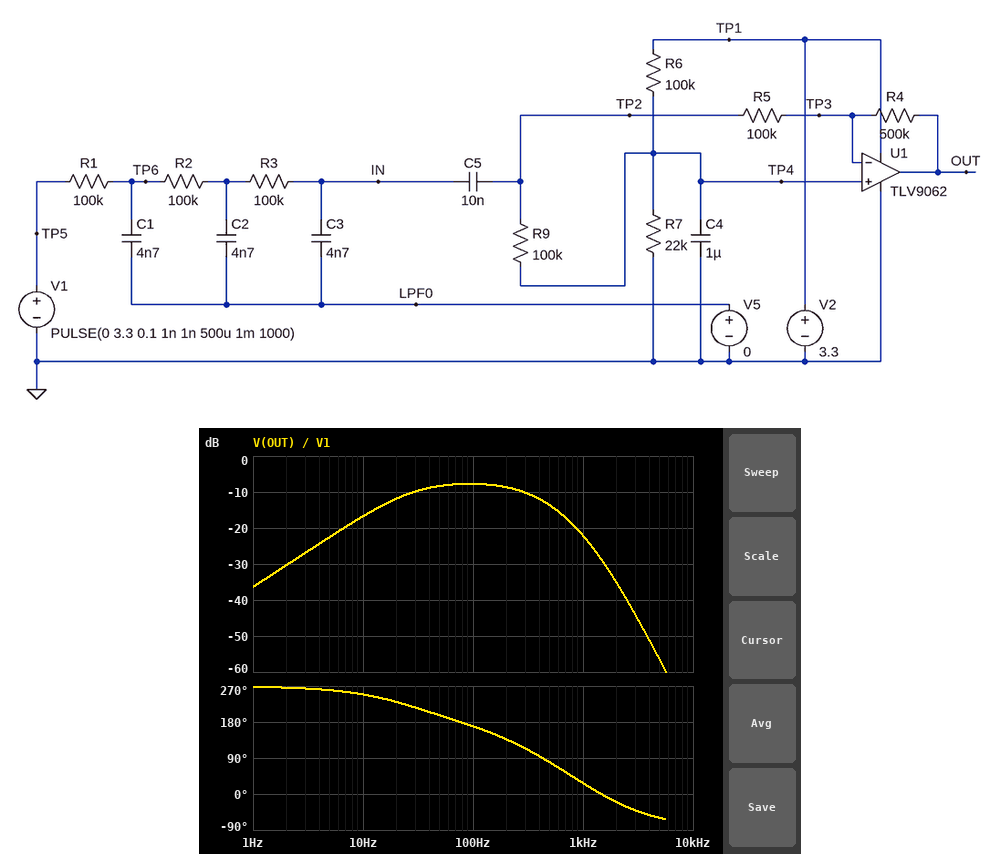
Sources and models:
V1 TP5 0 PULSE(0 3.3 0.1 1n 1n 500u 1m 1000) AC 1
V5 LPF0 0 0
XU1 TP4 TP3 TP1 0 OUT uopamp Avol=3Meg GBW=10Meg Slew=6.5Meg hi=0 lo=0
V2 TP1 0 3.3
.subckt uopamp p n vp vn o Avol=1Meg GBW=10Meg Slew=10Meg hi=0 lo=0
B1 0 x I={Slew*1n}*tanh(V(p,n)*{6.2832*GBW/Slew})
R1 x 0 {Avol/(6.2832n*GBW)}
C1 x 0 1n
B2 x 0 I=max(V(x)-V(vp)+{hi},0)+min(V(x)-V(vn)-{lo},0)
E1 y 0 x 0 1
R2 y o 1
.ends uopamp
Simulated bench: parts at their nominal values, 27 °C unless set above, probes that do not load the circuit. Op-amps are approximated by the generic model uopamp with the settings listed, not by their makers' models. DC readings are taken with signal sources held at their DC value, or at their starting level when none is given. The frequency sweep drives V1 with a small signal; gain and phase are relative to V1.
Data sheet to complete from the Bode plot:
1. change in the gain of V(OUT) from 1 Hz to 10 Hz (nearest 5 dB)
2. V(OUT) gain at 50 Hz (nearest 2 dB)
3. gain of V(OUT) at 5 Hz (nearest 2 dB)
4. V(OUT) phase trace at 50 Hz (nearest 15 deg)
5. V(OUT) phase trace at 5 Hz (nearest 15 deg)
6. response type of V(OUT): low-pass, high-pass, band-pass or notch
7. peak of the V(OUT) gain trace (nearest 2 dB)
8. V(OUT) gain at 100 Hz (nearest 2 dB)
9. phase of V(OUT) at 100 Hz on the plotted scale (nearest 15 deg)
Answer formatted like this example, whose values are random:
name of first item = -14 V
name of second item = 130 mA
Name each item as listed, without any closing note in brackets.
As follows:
change in the gain of V(OUT) from 1 Hz to 10 Hz = 20 dB
V(OUT) gain at 50 Hz = -8 dB
gain of V(OUT) at 5 Hz = -22 dB
V(OUT) phase trace at 50 Hz = 195 deg
V(OUT) phase trace at 5 Hz = 255 deg
response type of V(OUT): low-pass, high-pass, band-pass or notch = band-pass
peak of the V(OUT) gain trace = -8 dB
V(OUT) gain at 100 Hz = -8 dB
phase of V(OUT) at 100 Hz on the plotted scale = 165 deg
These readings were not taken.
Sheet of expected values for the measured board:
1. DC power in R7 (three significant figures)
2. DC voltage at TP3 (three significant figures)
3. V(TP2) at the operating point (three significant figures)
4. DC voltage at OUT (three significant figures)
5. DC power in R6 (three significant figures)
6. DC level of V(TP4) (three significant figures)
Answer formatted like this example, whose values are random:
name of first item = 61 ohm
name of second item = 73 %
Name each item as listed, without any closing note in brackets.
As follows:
DC power in R7 = 16.1 µW
DC voltage at TP3 = 595 mV
V(TP2) at the operating point = 595 mV
DC voltage at OUT = 595 mV
DC power in R6 = 73.2 µW
DC level of V(TP4) = 595 mV
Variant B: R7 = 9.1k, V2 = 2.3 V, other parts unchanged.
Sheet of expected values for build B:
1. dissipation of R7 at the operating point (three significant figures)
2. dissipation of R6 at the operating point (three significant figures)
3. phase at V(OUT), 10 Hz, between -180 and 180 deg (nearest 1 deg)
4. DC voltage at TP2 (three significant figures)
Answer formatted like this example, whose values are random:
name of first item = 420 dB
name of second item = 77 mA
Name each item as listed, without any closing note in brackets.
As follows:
dissipation of R7 at the operating point = 4.04 µW
dissipation of R6 at the operating point = 44.4 µW
phase at V(OUT), 10 Hz, between -180 and 180 deg = -112 deg
DC voltage at TP2 = 192 mV
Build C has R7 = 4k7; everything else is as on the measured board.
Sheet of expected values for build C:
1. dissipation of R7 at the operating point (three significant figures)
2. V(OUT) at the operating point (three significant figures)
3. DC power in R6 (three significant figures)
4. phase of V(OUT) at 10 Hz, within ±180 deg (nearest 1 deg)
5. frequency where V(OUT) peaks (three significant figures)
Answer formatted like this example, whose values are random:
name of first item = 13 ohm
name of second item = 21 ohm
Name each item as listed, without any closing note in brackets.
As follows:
dissipation of R7 at the operating point = 4.67 µW
V(OUT) at the operating point = 148 mV
DC power in R6 = 99.3 µW
phase of V(OUT) at 10 Hz, within ±180 deg = -112 deg
frequency where V(OUT) peaks = 93.8 Hz
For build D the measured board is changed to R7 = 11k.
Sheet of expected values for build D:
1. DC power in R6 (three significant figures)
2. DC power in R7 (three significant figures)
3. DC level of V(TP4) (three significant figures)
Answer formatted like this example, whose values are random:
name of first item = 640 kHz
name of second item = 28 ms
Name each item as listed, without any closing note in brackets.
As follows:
DC power in R6 = 88.4 µW
DC power in R7 = 9.72 µW
DC level of V(TP4) = 327 mV
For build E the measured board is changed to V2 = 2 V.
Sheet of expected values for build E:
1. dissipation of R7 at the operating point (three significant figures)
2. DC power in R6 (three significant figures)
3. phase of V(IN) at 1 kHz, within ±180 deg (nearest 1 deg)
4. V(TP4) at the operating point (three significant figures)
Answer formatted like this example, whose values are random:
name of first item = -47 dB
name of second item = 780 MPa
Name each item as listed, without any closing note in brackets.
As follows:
dissipation of R7 at the operating point = 5.91 µW
DC power in R6 = 26.9 µW
phase of V(IN) at 1 kHz, within ±180 deg = -170 deg
V(TP4) at the operating point = 361 mV
